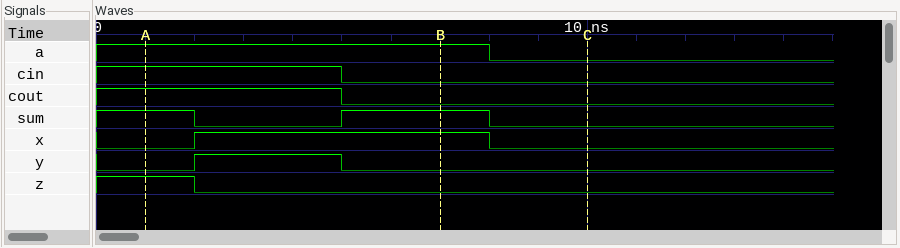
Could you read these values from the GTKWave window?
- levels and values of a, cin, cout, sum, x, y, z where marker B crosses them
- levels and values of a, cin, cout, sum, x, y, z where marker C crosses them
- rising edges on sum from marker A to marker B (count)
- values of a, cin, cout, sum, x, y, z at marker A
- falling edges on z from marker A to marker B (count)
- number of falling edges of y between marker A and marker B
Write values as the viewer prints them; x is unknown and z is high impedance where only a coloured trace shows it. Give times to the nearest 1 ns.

a=1, cin=0, cout=0, sum=1, x=1, y=0, z=0
a=0, cin=0, cout=0, sum=0, x=0, y=0, z=0
1
a=1, cin=1, cout=1, sum=1, x=0, y=0, z=1
1
1
